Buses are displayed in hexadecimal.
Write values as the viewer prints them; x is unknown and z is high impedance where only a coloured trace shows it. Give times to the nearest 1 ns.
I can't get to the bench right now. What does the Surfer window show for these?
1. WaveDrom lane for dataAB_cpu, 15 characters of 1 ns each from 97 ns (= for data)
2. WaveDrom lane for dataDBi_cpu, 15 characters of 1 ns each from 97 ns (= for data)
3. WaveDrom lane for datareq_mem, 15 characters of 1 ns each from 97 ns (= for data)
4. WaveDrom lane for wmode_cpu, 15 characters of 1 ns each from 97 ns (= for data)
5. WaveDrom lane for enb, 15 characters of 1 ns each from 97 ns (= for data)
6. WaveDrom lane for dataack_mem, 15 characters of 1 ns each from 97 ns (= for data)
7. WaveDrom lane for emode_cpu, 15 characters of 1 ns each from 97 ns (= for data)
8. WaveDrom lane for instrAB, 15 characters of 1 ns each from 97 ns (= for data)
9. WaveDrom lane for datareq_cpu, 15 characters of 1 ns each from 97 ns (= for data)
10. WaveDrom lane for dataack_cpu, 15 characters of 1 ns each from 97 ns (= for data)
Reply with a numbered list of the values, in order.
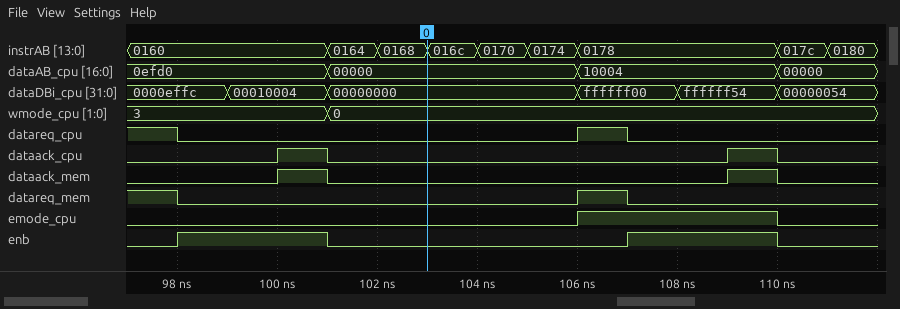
1. {name: 'dataAB_cpu', wave: '=...=....=...=.', data: '0efd0 00000 10004 00000'}
2. {name: 'dataDBi_cpu', wave: '=.=.=....=.=.=.', data: '0000effc 00010004 00000000 ffffff00 ffffff54 00000054'}
3. {name: 'datareq_mem', wave: '10.......10....'}
4. {name: 'wmode_cpu', wave: '=...=..........', data: '3 0'}
5. {name: 'enb', wave: '01..0.....1..0.'}
6. {name: 'dataack_mem', wave: '0..10.......10.'}
7. {name: 'emode_cpu', wave: '0........1...0.'}
8. {name: 'instrAB', wave: '=...======...==', data: '0160 0164 0168 016c 0170 0174 0178 017c 0180'}
9. {name: 'datareq_cpu', wave: '10.......10....'}
10. {name: 'dataack_cpu', wave: '0..10.......10.'}
